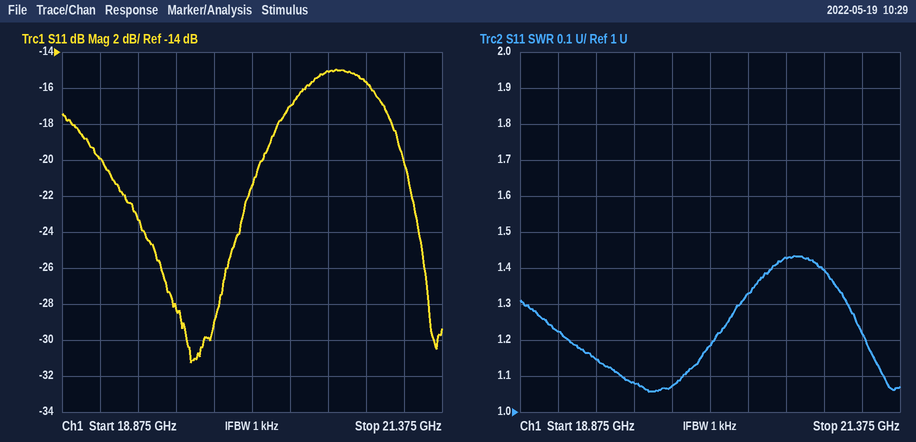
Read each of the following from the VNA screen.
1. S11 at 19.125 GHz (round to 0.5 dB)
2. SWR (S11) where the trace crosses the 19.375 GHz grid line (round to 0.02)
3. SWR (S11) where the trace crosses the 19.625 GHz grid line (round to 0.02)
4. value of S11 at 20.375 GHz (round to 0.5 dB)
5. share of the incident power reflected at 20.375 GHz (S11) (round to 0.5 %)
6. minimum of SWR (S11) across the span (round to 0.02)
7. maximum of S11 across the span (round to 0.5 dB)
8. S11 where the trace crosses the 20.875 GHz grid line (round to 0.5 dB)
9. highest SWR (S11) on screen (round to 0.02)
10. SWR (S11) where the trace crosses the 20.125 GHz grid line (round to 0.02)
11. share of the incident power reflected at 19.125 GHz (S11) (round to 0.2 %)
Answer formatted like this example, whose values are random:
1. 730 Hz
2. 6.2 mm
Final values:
1. -20.0 dB
2. 1.14
3. 1.08
4. -17.0 dB
5. 2.0 %
6. 1.06
7. -15.0 dB
8. -15.5 dB
9. 1.44
10. 1.18
11. 1.0 %
